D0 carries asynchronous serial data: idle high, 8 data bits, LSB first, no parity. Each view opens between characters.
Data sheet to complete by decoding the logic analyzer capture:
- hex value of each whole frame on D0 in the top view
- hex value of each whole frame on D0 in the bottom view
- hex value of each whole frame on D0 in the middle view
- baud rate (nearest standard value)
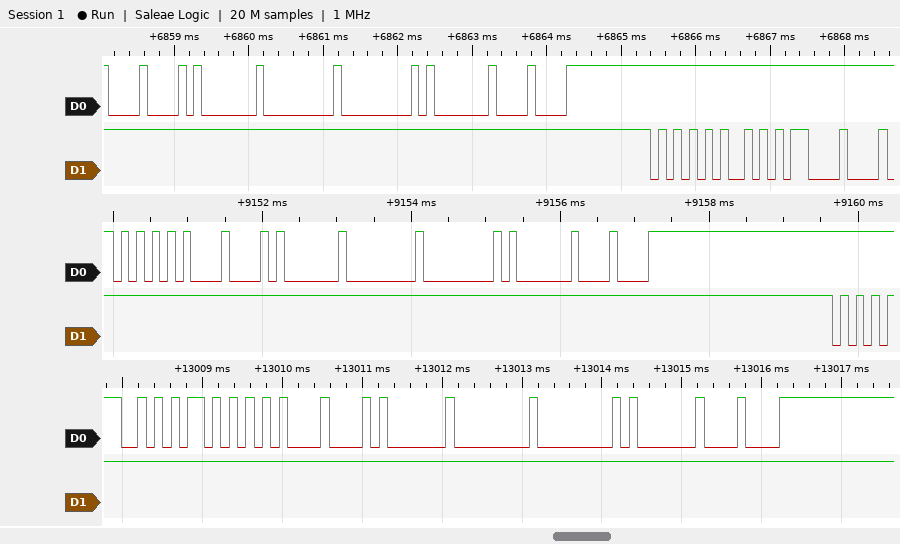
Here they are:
08, 01, 00, 00, 01, 08
AA, 55, 08, 01, 00, 00, 01, 08
55, 08, 01, 00, 00, 01, 08
9600 baud
